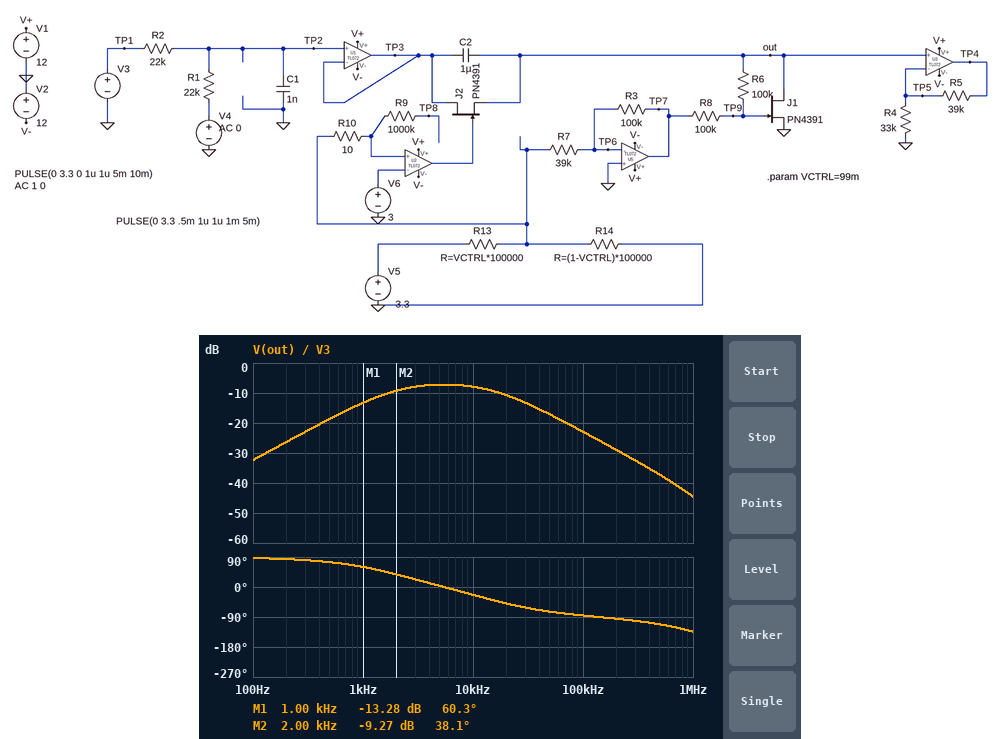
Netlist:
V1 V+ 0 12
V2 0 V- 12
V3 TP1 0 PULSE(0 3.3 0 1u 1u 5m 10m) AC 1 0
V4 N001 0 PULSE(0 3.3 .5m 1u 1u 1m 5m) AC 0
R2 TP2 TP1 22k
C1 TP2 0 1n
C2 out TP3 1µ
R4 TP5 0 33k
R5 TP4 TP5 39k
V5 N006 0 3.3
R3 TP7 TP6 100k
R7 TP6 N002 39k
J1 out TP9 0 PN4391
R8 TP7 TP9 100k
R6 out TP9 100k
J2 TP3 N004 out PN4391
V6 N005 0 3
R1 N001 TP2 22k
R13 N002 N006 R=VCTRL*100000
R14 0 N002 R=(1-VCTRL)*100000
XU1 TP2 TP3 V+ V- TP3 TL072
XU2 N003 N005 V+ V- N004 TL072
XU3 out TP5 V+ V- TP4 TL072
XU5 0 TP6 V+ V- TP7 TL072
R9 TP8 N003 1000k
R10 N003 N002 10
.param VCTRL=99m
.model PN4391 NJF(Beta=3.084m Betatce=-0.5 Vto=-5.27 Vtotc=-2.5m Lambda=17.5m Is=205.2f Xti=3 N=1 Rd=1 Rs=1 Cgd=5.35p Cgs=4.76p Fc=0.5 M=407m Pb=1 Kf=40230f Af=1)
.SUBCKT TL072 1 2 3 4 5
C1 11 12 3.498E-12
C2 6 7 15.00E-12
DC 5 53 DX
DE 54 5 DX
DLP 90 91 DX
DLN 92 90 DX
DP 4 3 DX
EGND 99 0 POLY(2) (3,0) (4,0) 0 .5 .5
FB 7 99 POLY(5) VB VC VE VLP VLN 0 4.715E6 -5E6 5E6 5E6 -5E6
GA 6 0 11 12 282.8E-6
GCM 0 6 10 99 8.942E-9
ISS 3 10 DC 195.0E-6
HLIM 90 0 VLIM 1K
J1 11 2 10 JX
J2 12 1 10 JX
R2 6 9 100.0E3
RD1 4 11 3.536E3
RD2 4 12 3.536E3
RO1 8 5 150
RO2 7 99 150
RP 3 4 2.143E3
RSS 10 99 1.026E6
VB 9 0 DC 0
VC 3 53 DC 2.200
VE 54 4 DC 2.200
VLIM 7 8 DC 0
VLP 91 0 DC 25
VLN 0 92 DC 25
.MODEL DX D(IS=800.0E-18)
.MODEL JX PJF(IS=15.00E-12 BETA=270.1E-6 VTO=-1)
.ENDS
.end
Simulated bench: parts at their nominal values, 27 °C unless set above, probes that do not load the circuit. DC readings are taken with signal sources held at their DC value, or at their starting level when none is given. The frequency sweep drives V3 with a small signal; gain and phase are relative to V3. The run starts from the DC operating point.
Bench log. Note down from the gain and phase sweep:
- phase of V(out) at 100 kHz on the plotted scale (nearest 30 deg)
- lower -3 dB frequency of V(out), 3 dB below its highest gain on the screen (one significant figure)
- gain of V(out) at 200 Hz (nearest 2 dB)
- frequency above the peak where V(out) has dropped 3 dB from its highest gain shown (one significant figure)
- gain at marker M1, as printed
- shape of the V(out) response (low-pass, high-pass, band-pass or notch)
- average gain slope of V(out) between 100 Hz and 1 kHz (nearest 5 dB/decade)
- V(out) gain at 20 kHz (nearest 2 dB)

-90 deg
2 kHz
-26 dB
20 kHz
-13.28 dB
band-pass
20 dB/decade
-10 dB
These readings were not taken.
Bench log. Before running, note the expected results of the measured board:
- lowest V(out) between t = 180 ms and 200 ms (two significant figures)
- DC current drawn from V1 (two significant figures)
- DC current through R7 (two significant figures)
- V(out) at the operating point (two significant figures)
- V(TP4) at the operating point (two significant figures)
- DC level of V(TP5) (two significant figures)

-1.2 V
46 mA
62 µA
-2.4 mV
-5.2 mV
-2.4 mV
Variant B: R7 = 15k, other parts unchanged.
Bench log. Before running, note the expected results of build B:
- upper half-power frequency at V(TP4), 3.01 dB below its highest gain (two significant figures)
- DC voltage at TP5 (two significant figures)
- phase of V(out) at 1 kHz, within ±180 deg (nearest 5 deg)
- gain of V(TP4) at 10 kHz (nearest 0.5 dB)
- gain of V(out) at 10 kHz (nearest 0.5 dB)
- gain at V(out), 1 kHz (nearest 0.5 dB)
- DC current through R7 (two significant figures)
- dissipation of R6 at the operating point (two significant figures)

15 kHz
-180 mV
0 deg
-1.0 dB
-7.5 dB
-6.0 dB
110 µA
260 µW
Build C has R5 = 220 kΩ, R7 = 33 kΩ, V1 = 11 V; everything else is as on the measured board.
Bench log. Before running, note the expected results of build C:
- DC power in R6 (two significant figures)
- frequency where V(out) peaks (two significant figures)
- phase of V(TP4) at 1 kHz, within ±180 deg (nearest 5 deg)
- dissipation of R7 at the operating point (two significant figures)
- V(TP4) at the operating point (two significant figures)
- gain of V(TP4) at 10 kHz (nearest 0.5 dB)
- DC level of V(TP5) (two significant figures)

130 µW
4.9 kHz
55 deg
170 µW
-26 mV
10.0 dB
-3.4 mV
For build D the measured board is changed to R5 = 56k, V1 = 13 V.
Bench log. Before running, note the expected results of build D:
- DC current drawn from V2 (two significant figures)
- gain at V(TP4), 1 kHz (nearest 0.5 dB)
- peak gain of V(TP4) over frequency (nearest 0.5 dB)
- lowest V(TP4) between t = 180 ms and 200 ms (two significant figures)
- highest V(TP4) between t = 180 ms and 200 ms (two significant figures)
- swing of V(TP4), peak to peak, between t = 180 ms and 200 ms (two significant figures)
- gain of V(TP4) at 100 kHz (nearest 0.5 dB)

47 mA
-4.5 dB
1.5 dB
-3.2 V
3.2 V
6.4 V
-14.5 dB
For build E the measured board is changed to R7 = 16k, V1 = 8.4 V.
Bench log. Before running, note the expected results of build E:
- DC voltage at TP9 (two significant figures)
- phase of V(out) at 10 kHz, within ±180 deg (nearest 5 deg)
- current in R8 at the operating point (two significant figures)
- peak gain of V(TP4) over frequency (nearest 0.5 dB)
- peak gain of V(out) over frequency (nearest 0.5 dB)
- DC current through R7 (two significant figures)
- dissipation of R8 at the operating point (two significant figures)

-5.3 V
-35 deg
51 µA
0.5 dB
-6.0 dB
110 µA
260 µW
